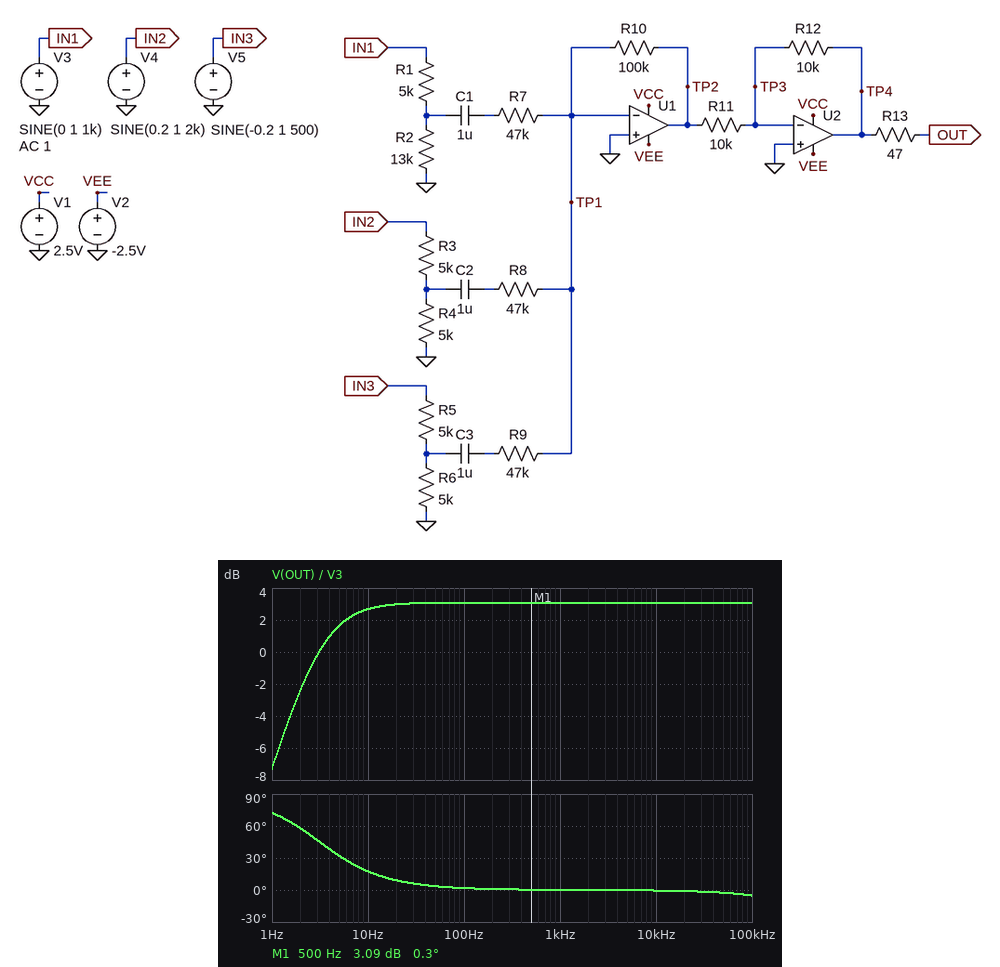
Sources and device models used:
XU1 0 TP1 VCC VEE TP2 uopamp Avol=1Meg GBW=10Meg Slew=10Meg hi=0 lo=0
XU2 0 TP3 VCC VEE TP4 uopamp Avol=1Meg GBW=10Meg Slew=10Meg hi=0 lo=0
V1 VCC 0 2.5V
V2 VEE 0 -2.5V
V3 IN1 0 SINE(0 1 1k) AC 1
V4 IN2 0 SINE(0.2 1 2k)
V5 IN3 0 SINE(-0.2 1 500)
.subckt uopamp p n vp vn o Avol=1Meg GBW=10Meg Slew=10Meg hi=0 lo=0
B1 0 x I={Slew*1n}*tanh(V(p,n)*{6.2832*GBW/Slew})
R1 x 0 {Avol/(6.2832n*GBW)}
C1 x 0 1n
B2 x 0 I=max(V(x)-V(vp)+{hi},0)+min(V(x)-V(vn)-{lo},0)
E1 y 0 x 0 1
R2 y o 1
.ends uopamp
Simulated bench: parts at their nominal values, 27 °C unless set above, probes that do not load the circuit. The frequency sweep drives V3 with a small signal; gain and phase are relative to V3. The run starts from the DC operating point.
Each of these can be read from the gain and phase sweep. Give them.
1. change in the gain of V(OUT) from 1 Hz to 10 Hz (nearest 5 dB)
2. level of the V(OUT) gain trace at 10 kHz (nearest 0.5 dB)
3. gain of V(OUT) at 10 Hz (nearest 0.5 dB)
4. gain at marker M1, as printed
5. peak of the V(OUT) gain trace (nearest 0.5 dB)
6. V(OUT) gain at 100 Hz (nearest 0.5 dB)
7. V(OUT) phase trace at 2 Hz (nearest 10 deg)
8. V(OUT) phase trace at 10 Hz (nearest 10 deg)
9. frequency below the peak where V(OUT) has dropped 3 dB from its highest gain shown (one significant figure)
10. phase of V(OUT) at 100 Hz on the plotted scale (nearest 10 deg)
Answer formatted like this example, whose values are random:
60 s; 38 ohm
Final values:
10 dB; 3.0 dB; 2.5 dB; 3.09 dB; 3.0 dB; 3.0 dB; 60 deg; 20 deg; 3 Hz; 0 deg
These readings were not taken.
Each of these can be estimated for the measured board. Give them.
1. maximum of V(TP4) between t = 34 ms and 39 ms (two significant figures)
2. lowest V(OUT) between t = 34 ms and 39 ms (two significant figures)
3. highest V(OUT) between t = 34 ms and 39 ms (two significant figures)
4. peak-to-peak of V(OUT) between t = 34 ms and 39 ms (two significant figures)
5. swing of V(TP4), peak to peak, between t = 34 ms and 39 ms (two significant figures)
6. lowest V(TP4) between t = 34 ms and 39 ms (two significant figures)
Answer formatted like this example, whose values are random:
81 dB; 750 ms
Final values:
2.5 V; -2.5 V; 2.5 V; 5.0 V; 5.0 V; -2.5 V
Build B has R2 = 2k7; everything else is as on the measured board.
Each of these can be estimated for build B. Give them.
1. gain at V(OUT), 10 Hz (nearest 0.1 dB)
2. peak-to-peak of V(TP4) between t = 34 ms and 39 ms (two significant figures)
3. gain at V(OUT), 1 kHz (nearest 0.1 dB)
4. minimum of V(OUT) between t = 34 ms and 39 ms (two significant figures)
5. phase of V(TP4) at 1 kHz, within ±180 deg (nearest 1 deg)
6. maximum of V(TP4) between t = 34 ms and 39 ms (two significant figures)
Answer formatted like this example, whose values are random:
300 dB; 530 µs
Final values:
-3.3 dB; 4.0 V; -2.9 dB; -2.0 V; 0 deg; 2.0 V
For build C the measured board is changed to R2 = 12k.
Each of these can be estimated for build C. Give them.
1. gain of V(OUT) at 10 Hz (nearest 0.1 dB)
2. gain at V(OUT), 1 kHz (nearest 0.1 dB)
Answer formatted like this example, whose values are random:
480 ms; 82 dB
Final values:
2.5 dB; 2.9 dB
